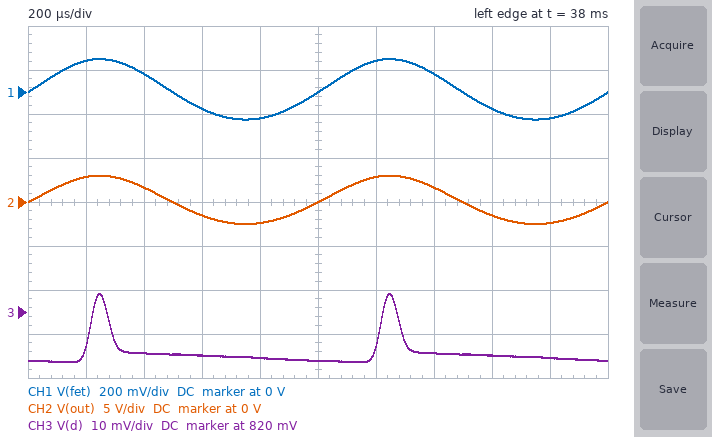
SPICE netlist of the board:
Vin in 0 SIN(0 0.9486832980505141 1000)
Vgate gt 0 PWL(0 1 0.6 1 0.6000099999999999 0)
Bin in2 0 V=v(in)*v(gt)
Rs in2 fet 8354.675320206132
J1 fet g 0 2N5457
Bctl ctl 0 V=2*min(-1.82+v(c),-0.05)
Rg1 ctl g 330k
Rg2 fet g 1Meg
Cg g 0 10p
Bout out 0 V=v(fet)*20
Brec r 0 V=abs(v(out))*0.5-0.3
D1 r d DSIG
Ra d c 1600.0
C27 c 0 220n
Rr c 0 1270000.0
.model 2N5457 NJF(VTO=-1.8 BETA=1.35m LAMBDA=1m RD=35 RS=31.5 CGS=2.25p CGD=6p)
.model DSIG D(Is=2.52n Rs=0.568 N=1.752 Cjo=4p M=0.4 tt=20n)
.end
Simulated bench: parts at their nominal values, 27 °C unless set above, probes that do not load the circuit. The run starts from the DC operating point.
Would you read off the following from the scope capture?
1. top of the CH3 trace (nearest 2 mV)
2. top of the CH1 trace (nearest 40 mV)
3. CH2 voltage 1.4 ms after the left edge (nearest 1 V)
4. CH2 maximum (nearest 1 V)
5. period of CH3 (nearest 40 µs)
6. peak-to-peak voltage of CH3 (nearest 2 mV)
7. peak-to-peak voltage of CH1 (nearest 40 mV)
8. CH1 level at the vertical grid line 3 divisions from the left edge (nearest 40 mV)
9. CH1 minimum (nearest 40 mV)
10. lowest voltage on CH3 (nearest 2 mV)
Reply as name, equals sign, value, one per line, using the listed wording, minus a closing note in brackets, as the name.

top of the CH3 trace = 824 mV
top of the CH1 trace = 160 mV
CH2 voltage 1.4 ms after the left edge = 2 V
CH2 maximum = 3 V
period of CH3 = 1.00 ms
peak-to-peak voltage of CH3 = 16 mV
peak-to-peak voltage of CH1 = 280 mV
CH1 level at the vertical grid line 3 divisions from the left edge = -80 mV
CH1 minimum = -120 mV
lowest voltage on CH3 = 808 mV
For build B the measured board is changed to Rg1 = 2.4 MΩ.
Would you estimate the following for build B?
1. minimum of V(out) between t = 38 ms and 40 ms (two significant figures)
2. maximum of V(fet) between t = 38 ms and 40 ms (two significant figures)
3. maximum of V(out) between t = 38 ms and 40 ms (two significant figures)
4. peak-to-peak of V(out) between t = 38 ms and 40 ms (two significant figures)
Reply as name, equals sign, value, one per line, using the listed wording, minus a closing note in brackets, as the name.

minimum of V(out) between t = 38 ms and 40 ms = -1.2 V
maximum of V(fet) between t = 38 ms and 40 ms = 58 mV
maximum of V(out) between t = 38 ms and 40 ms = 1.2 V
peak-to-peak of V(out) between t = 38 ms and 40 ms = 2.4 V
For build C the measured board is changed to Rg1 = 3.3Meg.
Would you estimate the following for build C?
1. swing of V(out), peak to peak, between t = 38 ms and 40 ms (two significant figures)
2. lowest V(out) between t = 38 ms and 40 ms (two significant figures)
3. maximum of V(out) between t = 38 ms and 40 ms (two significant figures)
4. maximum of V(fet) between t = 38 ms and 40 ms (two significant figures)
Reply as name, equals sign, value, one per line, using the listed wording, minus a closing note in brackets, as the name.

swing of V(out), peak to peak, between t = 38 ms and 40 ms = 2.0 V
lowest V(out) between t = 38 ms and 40 ms = -1.0 V
maximum of V(out) between t = 38 ms and 40 ms = 960 mV
maximum of V(fet) between t = 38 ms and 40 ms = 48 mV
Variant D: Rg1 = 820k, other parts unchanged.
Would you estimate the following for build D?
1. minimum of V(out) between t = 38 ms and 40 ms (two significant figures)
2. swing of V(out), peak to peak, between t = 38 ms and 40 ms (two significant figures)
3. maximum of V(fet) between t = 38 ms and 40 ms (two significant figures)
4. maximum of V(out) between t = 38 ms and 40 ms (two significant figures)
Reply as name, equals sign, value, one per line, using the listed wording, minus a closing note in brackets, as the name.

minimum of V(out) between t = 38 ms and 40 ms = -2.2 V
swing of V(out), peak to peak, between t = 38 ms and 40 ms = 4.5 V
maximum of V(fet) between t = 38 ms and 40 ms = 110 mV
maximum of V(out) between t = 38 ms and 40 ms = 2.2 V
